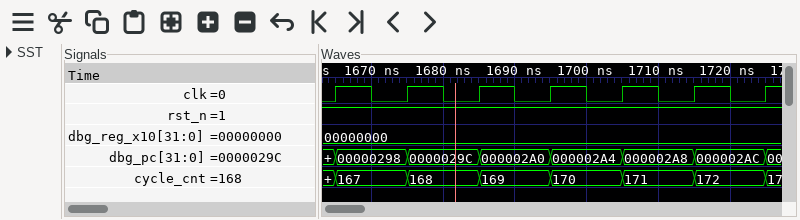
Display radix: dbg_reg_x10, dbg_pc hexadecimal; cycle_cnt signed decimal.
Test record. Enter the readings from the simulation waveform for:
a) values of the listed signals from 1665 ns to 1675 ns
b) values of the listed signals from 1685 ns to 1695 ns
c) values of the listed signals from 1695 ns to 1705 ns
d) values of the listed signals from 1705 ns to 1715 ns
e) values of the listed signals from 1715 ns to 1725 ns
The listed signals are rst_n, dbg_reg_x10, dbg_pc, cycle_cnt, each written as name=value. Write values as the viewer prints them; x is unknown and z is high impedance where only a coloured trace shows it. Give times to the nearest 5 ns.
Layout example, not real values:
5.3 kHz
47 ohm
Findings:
rst_n=1, dbg_reg_x10=00000000, dbg_pc=00000298, cycle_cnt=167
rst_n=1, dbg_reg_x10=00000000, dbg_pc=000002A0, cycle_cnt=169
rst_n=1, dbg_reg_x10=00000000, dbg_pc=000002A4, cycle_cnt=170
rst_n=1, dbg_reg_x10=00000000, dbg_pc=000002A8, cycle_cnt=171
rst_n=1, dbg_reg_x10=00000000, dbg_pc=000002AC, cycle_cnt=172
